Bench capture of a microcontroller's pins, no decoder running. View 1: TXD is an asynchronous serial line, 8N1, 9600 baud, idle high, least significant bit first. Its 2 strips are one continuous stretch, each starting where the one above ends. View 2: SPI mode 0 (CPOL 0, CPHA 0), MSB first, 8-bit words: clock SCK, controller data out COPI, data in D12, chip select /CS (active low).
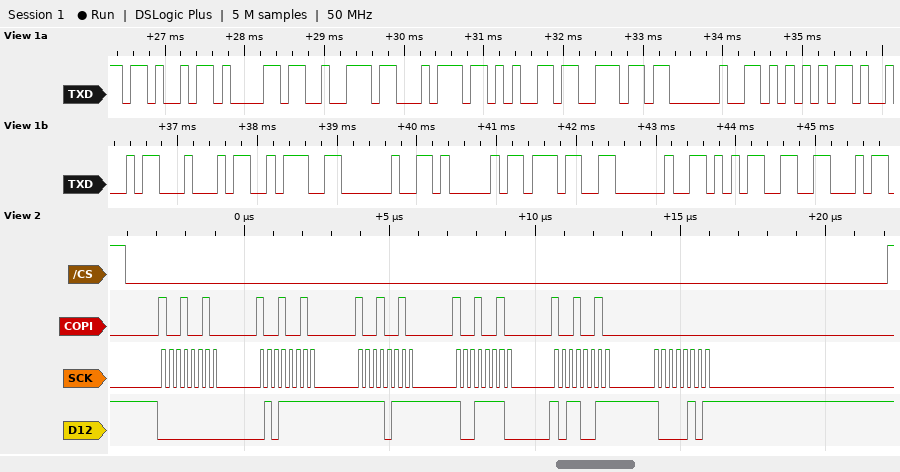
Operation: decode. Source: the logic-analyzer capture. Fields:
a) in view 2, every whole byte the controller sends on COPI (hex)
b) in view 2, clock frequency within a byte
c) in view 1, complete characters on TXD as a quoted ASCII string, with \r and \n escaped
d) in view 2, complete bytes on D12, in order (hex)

0x92 0x92 0x92 0x92 0x92 0x00
4 MHz
"Karten UID: A7 5F"
0x00 0x5F 0xF7 0x9E 0xB3 0x85
